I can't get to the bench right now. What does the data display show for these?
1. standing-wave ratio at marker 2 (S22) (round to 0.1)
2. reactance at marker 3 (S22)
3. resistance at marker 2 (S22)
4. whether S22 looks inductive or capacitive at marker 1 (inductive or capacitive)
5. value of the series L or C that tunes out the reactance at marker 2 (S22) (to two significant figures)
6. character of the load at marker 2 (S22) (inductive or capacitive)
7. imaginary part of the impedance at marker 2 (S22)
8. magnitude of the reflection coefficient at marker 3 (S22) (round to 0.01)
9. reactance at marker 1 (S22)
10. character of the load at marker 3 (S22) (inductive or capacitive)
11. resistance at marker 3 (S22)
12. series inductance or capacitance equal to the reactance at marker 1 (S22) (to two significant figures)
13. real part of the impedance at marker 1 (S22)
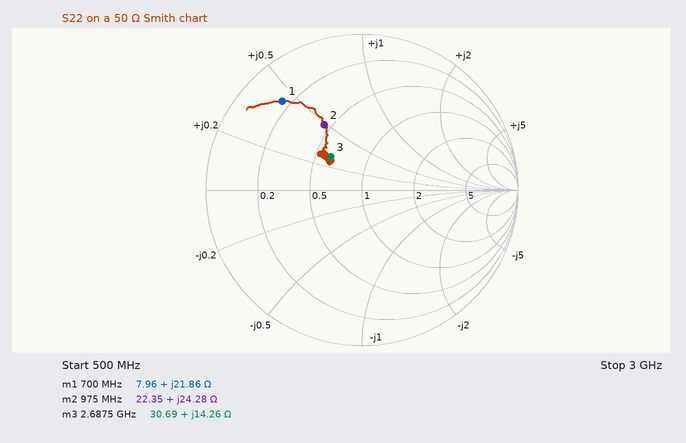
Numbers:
2.9
+14.26 Ω
22.35 Ω
inductive
6.7 pF
inductive
+24.28 Ω
0.29
+21.86 Ω
inductive
30.69 Ω
5.0 nH
7.96 Ω
